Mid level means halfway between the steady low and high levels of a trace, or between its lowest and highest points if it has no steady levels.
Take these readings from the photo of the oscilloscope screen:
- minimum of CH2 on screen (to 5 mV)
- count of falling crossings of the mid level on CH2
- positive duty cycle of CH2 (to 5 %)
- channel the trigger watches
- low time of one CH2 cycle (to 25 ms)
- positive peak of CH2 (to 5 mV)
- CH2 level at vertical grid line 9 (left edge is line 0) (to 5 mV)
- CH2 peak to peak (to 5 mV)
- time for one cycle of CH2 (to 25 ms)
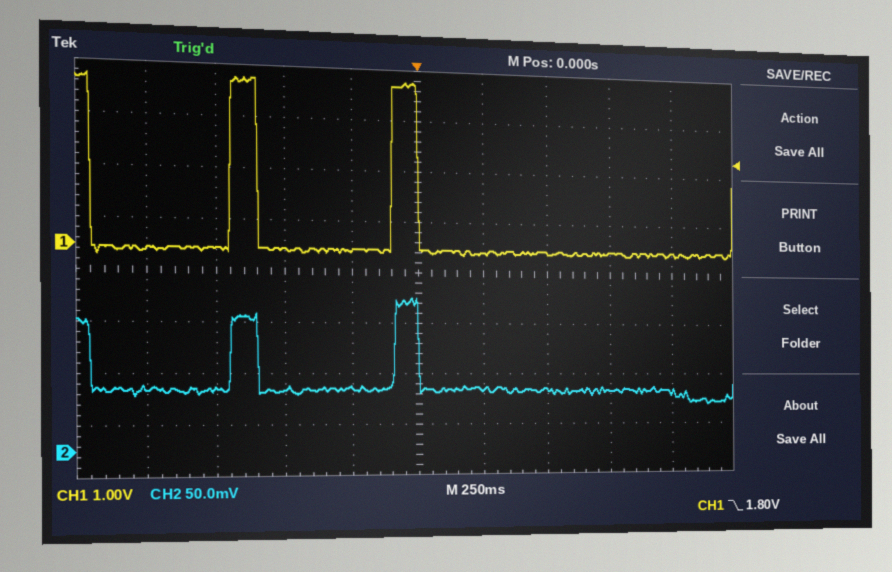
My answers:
45 mV
3
15 %
CH1
500 ms
150 mV
55 mV
105 mV
600 ms
